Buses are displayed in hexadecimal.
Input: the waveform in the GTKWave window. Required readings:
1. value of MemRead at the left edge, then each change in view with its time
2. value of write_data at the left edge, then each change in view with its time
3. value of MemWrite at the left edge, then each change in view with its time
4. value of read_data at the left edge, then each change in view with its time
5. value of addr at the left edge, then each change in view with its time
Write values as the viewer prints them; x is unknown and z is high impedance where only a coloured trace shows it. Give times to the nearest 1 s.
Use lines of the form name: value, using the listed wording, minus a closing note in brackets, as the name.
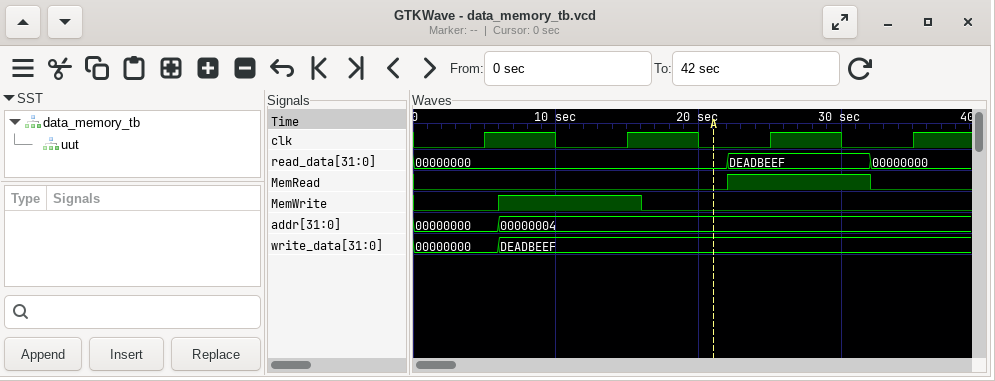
value of MemRead at the left edge, then each change in view with its time: 0, 1 at 22 s, 0 at 32 s
value of write_data at the left edge, then each change in view with its time: 00000000, DEADBEEF at 6 s
value of MemWrite at the left edge, then each change in view with its time: 0, 1 at 6 s, 0 at 16 s
value of read_data at the left edge, then each change in view with its time: 00000000, DEADBEEF at 22 s, 00000000 at 32 s
value of addr at the left edge, then each change in view with its time: 00000000, 00000004 at 6 s
